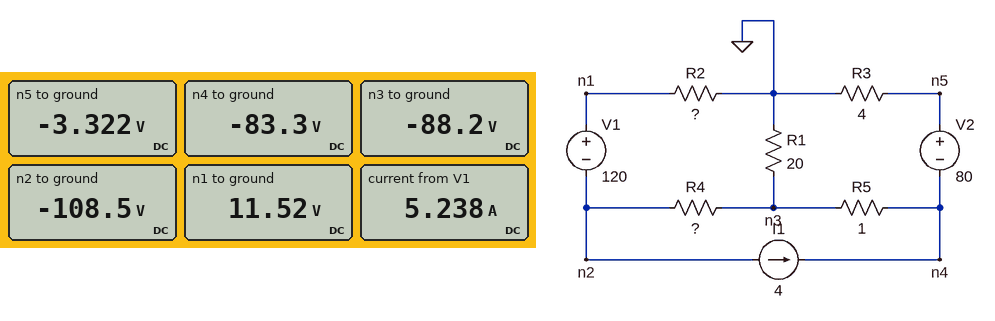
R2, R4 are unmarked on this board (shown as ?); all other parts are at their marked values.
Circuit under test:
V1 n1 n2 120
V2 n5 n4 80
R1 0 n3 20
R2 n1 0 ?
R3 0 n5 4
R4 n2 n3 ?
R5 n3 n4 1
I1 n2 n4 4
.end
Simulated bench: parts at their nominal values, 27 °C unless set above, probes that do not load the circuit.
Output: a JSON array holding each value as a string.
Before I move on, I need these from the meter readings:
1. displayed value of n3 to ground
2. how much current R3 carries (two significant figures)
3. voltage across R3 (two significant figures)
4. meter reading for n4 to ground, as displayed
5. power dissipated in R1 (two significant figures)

["-88.2 V", "830 mA", "3.3 V", "-83.3 V", "390 W"]
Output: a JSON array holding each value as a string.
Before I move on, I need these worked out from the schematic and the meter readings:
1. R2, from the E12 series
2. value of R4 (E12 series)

["2.2 Ω", "2.2 Ω"]
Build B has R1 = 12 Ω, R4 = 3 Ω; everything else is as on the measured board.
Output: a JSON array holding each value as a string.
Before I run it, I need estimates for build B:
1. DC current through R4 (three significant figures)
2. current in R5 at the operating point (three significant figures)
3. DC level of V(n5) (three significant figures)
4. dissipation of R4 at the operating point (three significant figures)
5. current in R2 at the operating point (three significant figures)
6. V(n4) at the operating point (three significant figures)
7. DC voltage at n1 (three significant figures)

["9.58 A", "3.00 A", "4.01 V", "275 W", "5.58 A", "-76.0 V", "12.3 V"]
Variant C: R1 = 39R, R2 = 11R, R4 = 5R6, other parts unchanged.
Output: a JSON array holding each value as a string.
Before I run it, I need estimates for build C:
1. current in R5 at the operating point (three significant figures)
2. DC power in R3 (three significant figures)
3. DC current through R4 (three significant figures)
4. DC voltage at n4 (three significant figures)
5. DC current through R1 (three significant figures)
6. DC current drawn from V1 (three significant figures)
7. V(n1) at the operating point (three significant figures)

["3.07 A", "3.49 W", "5.10 A", "-76.3 V", "2.03 A", "1.10 A", "12.1 V"]
